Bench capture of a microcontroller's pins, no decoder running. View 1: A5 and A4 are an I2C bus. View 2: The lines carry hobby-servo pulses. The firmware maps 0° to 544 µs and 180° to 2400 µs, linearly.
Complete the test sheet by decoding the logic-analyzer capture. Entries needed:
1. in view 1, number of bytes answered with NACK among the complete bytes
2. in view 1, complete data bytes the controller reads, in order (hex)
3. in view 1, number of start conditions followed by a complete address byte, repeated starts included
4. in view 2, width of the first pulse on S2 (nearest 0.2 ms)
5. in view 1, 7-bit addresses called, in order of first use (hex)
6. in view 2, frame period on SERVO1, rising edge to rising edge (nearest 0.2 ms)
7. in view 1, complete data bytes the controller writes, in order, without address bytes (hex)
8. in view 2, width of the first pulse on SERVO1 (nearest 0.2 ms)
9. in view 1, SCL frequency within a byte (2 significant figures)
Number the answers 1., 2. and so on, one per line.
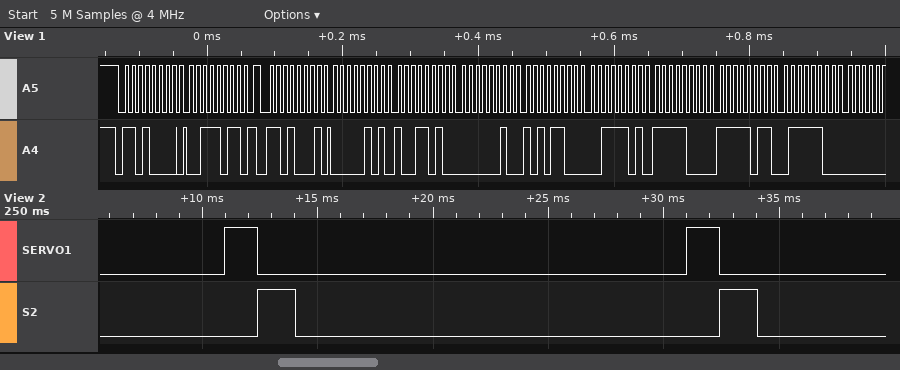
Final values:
1. 0
2. 05 9A 02 AC 3D F8 FB 7C
3. 2
4. 1.6 ms
5. 0x68
6. 20.0 ms
7. 3B
8. 1.4 ms
9. 100 kHz
